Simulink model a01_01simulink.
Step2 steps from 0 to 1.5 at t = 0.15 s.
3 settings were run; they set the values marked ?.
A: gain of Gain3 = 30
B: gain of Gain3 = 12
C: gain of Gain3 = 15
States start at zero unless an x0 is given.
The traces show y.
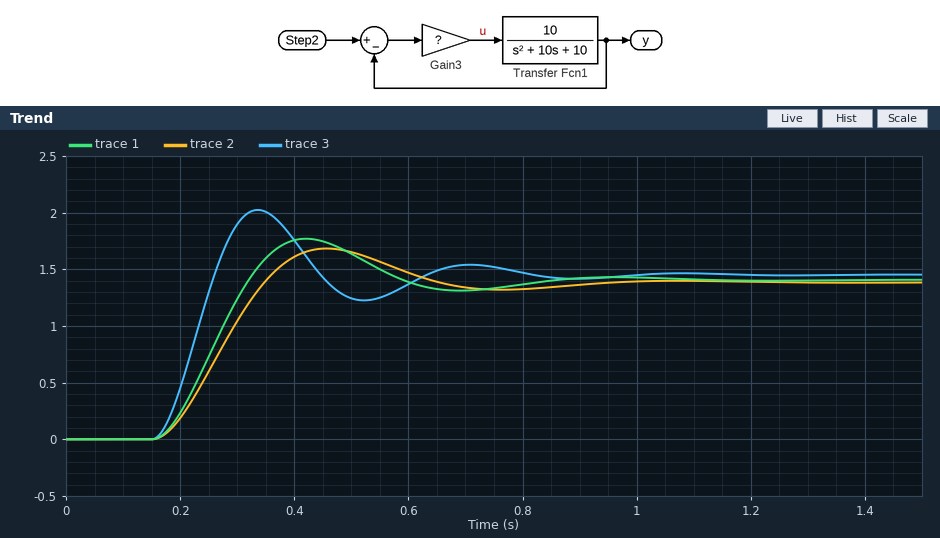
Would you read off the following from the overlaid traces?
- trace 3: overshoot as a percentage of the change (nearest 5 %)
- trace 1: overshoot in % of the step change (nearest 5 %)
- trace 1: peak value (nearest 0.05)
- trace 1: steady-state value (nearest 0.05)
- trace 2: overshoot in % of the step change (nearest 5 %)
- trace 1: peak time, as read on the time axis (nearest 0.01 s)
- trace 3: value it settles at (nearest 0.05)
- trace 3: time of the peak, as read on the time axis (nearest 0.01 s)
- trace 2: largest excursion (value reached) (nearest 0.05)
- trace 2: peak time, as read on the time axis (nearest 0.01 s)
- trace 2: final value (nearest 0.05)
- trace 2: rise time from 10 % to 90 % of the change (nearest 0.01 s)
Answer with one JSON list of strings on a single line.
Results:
["40 %", "25 %", "1.75", "1.40", "20 %", "0.42 s", "1.45", "0.34 s", "1.70", "0.46 s", "1.40", "0.13 s"]
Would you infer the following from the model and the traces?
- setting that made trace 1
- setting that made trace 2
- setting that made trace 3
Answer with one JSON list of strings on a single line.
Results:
["C", "B", "A"]
